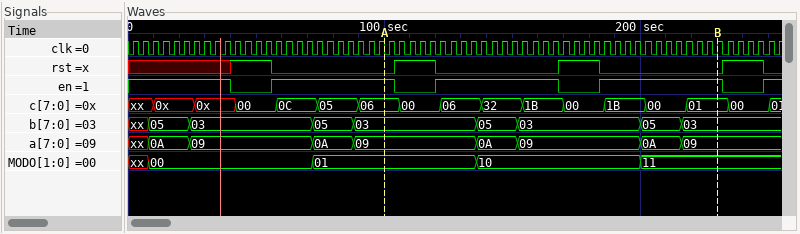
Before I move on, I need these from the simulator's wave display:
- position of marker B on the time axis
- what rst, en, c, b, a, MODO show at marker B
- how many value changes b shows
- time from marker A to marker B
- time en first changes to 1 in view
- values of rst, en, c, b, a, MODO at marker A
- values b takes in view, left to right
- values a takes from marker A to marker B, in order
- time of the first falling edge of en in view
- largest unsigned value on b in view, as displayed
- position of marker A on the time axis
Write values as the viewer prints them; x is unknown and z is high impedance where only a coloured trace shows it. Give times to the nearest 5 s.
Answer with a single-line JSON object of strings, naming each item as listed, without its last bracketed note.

{"position of marker B on the time axis": "230 s", "what rst, en, c, b, a, MODO show at marker B": "rst=0, en=1, c=01, b=03, a=09, MODO=11", "how many value changes b shows": "8", "time from marker A to marker B": "130 s", "time en first changes to 1 in view": "55 s", "values of rst, en, c, b, a, MODO at marker A": "rst=0, en=1, c=06, b=03, a=09, MODO=01", "values b takes in view, left to right": "xx, 05, 03, 05, 03, 05, 03, 05, 03", "values a takes from marker A to marker B, in order": "09, 0A, 09, 0A, 09", "time of the first falling edge of en in view": "40 s", "largest unsigned value on b in view, as displayed": "05", "position of marker A on the time axis": "100 s"}
